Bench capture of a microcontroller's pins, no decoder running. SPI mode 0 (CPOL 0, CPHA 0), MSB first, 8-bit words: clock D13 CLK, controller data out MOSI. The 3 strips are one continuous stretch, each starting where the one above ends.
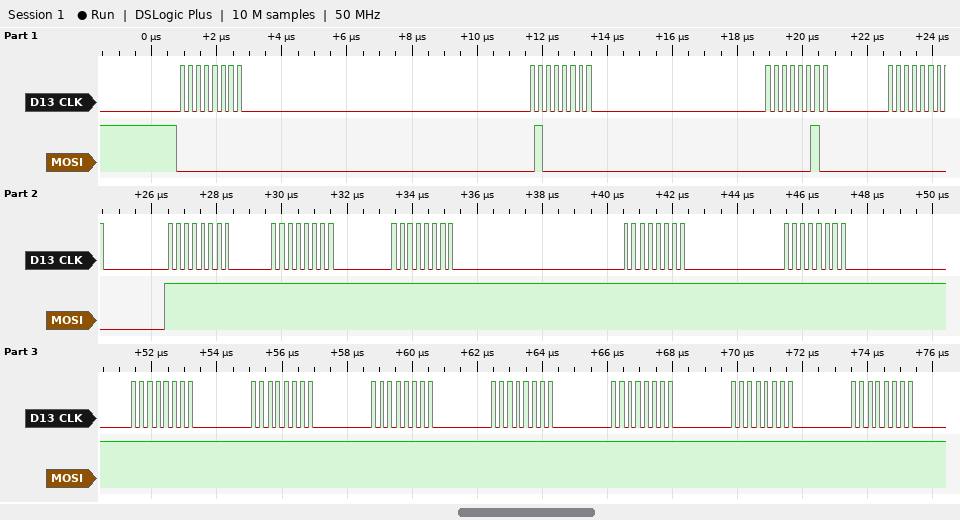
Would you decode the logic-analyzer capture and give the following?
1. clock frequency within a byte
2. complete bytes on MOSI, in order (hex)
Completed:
4 MHz
00 40 02 00 FF FF FF FF FF FF FF FF FF FF FF FF
